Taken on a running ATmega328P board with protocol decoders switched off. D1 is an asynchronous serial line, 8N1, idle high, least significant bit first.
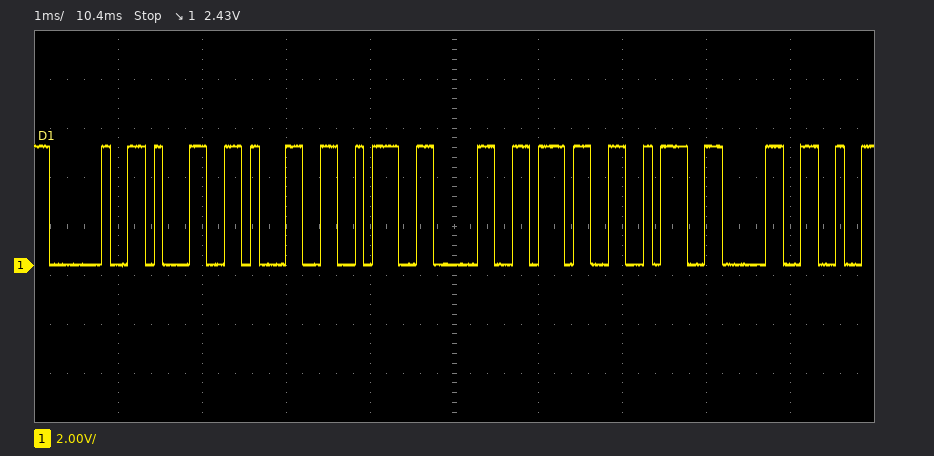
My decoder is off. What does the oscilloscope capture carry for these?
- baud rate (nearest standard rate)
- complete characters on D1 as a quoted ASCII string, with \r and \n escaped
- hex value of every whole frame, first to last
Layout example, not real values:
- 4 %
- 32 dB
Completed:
- 9600 baud
- " 11:07:0"
- 0x20 0x31 0x31 0x3A 0x30 0x37 0x3A 0x30
